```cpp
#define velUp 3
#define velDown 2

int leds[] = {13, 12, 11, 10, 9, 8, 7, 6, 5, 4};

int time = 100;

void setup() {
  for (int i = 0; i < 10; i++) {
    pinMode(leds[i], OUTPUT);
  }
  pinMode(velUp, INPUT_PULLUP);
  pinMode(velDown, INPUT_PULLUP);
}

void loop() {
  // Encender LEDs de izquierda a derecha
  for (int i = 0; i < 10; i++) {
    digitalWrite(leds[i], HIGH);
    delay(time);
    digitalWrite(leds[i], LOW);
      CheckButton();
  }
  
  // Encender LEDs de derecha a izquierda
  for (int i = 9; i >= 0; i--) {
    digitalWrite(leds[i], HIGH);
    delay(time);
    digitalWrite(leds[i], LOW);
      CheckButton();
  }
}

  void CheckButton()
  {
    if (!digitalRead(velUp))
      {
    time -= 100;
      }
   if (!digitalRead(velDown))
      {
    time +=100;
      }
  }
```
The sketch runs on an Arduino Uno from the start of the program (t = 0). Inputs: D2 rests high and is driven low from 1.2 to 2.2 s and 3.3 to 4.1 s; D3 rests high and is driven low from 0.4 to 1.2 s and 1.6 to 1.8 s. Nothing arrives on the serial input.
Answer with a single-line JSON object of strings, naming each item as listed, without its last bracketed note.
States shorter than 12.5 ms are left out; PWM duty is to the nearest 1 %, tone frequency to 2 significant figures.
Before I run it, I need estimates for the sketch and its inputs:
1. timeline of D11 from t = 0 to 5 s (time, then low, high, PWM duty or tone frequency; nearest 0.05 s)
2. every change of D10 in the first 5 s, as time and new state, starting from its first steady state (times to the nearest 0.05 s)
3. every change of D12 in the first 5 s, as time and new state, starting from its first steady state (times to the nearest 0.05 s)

{"timeline of D11 from t = 0 to 5 s": "0 s low; 0.2 s high; 0.3 s low", "every change of D10 in the first 5 s, as time and new state, starting from its first steady state": "0 s low; 0.3 s high; 0.4 s low", "every change of D12 in the first 5 s, as time and new state, starting from its first steady state": "0 s low; 0.1 s high; 0.2 s low"}
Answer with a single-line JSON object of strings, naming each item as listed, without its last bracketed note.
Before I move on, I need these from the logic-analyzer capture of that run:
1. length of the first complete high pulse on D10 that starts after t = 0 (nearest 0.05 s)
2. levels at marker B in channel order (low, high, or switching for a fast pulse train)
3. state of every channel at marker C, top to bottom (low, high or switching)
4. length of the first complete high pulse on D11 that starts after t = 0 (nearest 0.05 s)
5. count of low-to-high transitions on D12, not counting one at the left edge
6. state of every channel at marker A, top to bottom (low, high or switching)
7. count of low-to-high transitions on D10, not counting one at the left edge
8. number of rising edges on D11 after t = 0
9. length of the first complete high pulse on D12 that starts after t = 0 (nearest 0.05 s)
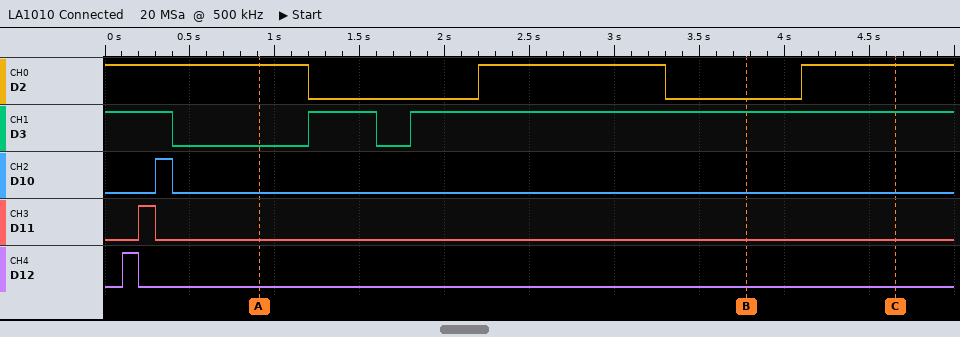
{"length of the first complete high pulse on D10 that starts after t = 0": "0.10 s", "levels at marker B in channel order": "D2 low, D3 high, D10 low, D11 low, D12 low", "state of every channel at marker C, top to bottom": "D2 high, D3 high, D10 low, D11 low, D12 low", "length of the first complete high pulse on D11 that starts after t = 0": "0.10 s", "count of low-to-high transitions on D12, not counting one at the left edge": "1", "state of every channel at marker A, top to bottom": "D2 high, D3 low, D10 low, D11 low, D12 low", "count of low-to-high transitions on D10, not counting one at the left edge": "1", "number of rising edges on D11 after t = 0": "1", "length of the first complete high pulse on D12 that starts after t = 0": "0.10 s"}
